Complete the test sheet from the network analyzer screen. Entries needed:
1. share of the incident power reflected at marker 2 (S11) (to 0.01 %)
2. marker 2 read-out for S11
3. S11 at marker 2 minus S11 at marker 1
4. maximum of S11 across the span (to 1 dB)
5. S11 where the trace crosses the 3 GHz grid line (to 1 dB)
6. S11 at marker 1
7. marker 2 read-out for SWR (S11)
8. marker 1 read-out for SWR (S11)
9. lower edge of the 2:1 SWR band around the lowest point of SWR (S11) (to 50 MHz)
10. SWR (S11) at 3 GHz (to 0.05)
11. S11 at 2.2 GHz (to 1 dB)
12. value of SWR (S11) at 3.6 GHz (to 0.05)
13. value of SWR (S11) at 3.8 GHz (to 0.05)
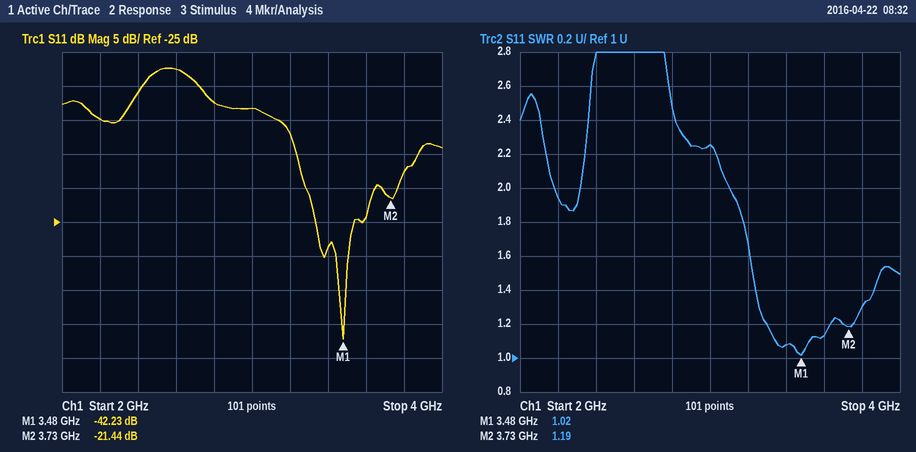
0.72 %
-21.44 dB
20.79 dB
-2 dB
-8 dB
-42.23 dB
1.19
1.02
3.10 GHz
2.25
-10 dB
1.15
1.30
